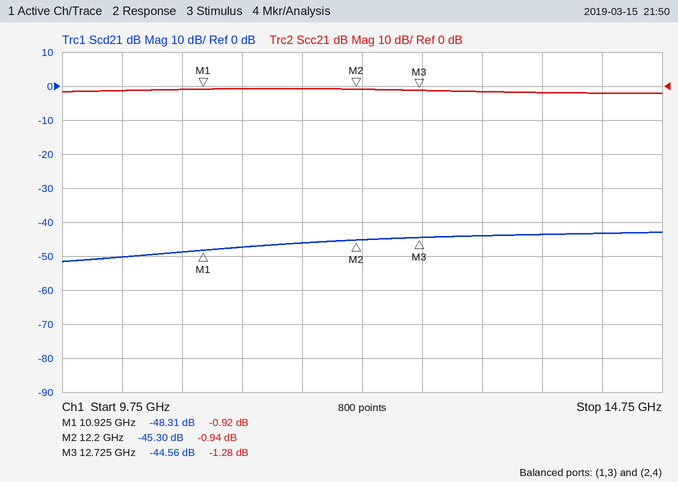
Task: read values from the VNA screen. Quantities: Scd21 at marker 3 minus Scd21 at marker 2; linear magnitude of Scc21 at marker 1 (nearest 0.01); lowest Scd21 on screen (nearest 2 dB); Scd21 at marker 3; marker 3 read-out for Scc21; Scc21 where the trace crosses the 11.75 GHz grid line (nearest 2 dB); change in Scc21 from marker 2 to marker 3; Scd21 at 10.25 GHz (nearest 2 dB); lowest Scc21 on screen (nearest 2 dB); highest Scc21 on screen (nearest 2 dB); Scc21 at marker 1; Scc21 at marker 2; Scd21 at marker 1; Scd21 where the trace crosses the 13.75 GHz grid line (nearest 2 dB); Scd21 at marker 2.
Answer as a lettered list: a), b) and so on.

a) 0.74 dB
b) 0.90
c) -52 dB
d) -44.56 dB
e) -1.28 dB
f) 0 dB
g) -0.34 dB
h) -50 dB
i) -2 dB
j) 0 dB
k) -0.92 dB
l) -0.94 dB
m) -48.31 dB
n) -44 dB
o) -45.30 dB
